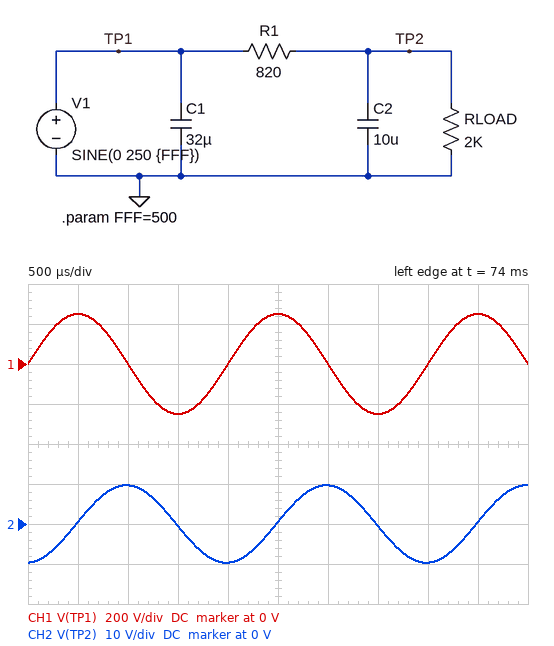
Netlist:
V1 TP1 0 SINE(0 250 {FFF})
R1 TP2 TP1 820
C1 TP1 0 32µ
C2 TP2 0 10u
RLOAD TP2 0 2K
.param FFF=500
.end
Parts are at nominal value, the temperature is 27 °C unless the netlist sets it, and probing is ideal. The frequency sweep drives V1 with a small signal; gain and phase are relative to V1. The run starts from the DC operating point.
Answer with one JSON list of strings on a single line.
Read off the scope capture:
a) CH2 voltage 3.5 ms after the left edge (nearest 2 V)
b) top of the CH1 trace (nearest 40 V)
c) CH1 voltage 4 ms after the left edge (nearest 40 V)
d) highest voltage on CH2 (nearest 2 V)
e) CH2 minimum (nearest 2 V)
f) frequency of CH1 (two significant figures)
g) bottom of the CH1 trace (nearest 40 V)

["0 V", "240 V", "0 V", "10 V", "-10 V", "500 Hz", "-240 V"]
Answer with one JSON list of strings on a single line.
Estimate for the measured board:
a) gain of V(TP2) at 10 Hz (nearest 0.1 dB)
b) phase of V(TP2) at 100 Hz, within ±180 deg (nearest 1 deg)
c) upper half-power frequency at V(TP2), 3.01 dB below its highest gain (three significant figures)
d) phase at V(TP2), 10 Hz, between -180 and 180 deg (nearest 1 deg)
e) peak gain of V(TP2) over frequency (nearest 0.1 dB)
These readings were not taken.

["-3.5 dB", "-75 deg", "27.4 Hz", "-20 deg", "-3.0 dB"]
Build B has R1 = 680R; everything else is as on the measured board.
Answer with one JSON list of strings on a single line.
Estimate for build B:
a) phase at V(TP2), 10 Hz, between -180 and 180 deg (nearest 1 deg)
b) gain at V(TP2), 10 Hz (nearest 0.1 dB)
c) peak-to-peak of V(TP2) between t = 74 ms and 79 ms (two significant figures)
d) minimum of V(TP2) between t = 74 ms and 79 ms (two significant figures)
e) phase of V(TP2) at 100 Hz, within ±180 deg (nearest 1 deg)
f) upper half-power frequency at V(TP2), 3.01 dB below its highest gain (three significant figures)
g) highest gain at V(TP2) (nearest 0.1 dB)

["-18 deg", "-3.0 dB", "23 V", "-12 V", "-73 deg", "31.4 Hz", "-2.5 dB"]
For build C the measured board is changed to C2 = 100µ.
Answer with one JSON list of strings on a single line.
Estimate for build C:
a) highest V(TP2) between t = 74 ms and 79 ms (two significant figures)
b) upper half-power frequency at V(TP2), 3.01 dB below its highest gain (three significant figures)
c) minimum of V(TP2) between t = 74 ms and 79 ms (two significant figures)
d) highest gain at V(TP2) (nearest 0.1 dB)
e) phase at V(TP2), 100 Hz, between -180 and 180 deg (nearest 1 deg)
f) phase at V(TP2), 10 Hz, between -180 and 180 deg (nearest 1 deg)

["1.2 V", "2.74 Hz", "-720 mV", "-3.0 dB", "-88 deg", "-75 deg"]
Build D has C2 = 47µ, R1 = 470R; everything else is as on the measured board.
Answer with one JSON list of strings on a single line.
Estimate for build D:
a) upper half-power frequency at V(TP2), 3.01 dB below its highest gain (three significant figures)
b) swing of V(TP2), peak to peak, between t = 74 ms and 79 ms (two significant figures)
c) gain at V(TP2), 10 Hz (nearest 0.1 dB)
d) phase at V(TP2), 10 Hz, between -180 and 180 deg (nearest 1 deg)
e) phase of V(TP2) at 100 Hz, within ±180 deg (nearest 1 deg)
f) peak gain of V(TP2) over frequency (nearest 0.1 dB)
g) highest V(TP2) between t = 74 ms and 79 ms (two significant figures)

["8.90 Hz", "7.2 V", "-5.4 dB", "-48 deg", "-85 deg", "-1.8 dB", "3.7 V"]
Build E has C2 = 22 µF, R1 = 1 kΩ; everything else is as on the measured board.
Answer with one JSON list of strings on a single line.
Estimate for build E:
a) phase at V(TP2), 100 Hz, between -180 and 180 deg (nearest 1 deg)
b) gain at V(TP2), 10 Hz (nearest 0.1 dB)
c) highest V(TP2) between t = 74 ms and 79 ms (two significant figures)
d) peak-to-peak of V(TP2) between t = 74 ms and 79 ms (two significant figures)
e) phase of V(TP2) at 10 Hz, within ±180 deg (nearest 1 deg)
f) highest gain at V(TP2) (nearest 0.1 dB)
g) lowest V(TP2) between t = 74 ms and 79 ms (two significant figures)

["-84 deg", "-6.2 dB", "3.6 V", "7.2 V", "-43 deg", "-3.5 dB", "-3.6 V"]
